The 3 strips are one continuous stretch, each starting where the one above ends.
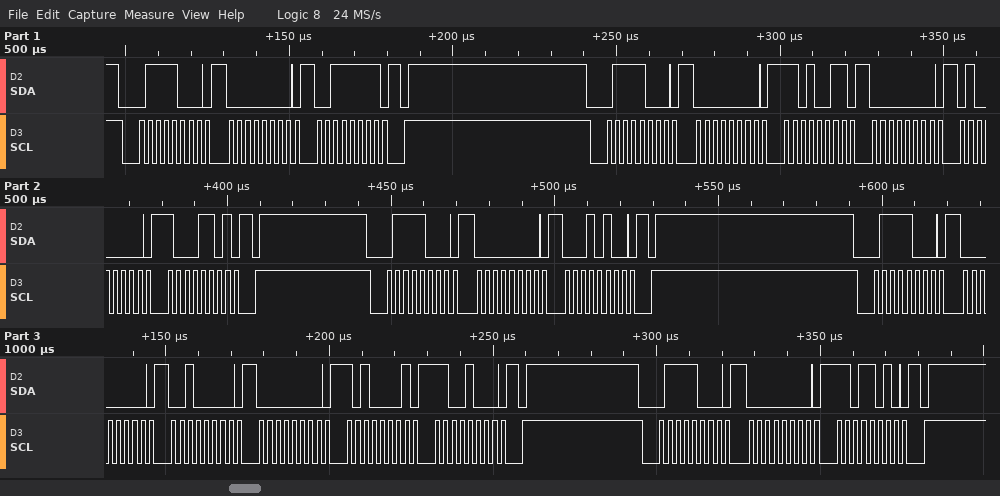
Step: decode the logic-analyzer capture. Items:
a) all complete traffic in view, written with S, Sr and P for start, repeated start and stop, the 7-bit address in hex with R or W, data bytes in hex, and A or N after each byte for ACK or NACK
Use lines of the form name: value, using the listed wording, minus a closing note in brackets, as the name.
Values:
all complete traffic in view, written with S, Sr and P for start, repeated start and stop, the 7-bit address in hex with R or W, data bytes in hex, and A or N after each byte for ACK or NACK: S 3CW A 00 A 3F A P S 3CW A 00 A D3 A 00 A 40 A 8D A P S 3CW A 00 A 14 A P S 3CW A 00 A 20 A 00 A A1 A C8 A P S 3CW A 00 A DA A P
